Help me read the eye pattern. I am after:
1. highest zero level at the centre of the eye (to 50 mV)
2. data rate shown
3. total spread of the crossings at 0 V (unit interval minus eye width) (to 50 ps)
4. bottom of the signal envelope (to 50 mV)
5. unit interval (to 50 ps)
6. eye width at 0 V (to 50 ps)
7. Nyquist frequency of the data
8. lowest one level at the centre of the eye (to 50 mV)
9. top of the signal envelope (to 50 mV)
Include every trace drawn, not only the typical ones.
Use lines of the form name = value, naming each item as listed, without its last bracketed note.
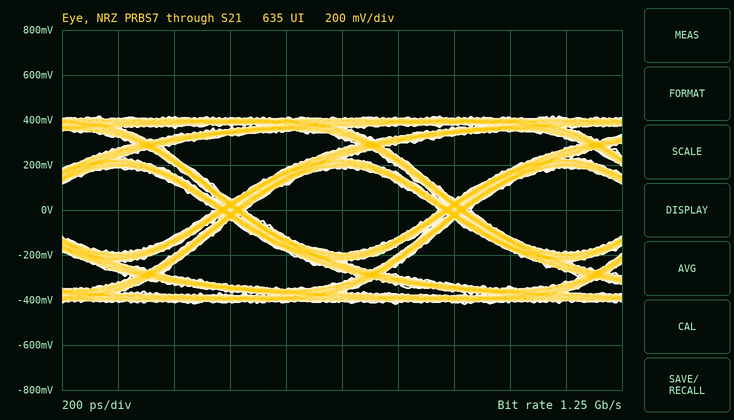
highest zero level at the centre of the eye = -200 mV
data rate shown = 1.25 Gb/s
total spread of the crossings at 0 V (unit interval minus eye width) = 100 ps
bottom of the signal envelope = -400 mV
unit interval = 800 ps
eye width at 0 V = 700 ps
Nyquist frequency of the data = 625 MHz
lowest one level at the centre of the eye = 200 mV
top of the signal envelope = 400 mV
